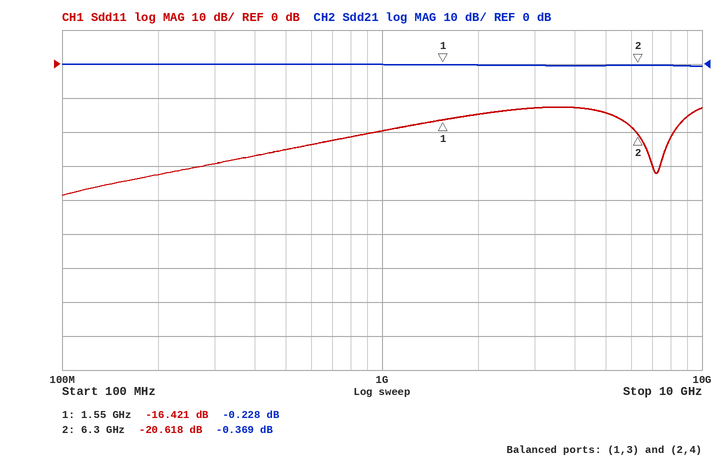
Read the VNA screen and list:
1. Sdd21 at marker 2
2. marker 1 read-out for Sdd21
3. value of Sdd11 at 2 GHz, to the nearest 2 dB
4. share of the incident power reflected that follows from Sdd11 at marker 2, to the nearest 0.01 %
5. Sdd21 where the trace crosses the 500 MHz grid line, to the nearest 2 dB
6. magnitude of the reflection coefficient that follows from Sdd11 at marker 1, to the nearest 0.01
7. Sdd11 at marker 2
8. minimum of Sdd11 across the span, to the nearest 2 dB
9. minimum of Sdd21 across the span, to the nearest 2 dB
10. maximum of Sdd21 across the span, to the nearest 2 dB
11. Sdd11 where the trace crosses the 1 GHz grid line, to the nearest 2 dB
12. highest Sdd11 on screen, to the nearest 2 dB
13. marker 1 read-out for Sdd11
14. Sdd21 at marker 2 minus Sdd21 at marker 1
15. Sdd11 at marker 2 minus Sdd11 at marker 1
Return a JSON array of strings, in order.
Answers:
["-0.369 dB", "-0.228 dB", "-14 dB", "0.87 %", "0 dB", "0.15", "-20.618 dB", "-38 dB", "0 dB", "0 dB", "-20 dB", "-12 dB", "-16.421 dB", "-0.141 dB", "-4.197 dB"]
